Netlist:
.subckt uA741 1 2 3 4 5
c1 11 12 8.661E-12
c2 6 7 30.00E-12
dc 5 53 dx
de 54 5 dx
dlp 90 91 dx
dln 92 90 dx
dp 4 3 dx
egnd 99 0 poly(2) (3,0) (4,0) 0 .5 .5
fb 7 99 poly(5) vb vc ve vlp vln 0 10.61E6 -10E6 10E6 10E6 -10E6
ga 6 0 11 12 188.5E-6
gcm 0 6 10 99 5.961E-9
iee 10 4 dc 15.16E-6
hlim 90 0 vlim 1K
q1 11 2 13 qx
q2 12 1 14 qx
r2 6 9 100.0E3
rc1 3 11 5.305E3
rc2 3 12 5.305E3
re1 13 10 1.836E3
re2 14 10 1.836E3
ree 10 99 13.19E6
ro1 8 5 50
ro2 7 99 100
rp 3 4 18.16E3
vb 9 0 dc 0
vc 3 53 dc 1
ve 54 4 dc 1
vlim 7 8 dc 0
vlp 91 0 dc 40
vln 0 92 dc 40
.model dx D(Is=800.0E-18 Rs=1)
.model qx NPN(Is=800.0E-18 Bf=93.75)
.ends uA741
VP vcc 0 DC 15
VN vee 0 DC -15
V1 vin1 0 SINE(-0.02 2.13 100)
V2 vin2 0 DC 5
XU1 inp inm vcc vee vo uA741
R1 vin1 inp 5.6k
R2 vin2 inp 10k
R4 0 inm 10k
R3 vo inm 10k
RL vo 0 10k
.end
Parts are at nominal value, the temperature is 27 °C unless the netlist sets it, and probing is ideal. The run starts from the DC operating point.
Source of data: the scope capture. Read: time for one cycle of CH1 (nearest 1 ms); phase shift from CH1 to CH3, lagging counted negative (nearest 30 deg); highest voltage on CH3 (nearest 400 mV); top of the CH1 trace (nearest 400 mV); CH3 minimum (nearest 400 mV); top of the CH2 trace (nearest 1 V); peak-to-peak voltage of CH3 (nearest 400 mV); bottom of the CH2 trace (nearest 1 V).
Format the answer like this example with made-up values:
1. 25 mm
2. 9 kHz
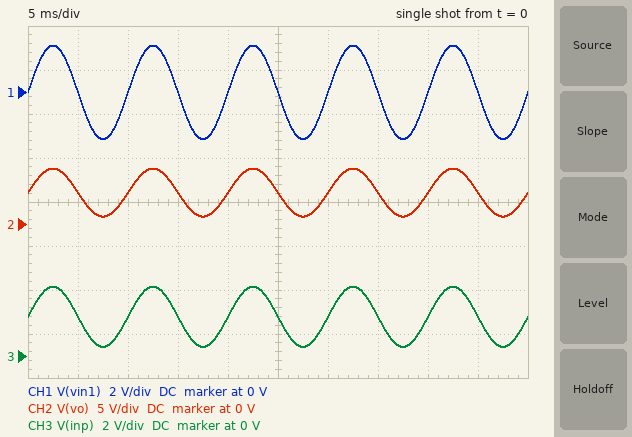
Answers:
1. 10 ms
2. 0 deg
3. 3.2 V
4. 2.0 V
5. 400 mV
6. 6 V
7. 2.8 V
8. 1 V
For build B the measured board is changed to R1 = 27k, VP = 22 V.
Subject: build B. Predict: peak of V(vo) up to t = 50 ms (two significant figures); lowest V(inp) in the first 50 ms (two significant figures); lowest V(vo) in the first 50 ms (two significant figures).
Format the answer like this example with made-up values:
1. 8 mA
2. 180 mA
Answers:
1. 8.4 V
2. 3.1 V
3. 6.1 V
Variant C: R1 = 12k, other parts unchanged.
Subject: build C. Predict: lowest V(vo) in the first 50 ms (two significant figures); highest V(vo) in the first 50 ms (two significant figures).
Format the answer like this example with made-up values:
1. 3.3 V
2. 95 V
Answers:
1. 3.5 V
2. 7.4 V
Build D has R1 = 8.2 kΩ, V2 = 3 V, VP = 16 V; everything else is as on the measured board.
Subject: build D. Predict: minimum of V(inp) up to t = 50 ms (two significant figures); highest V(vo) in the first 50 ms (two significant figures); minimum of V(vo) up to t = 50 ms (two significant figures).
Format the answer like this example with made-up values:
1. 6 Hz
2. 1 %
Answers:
1. 170 mV
2. 5.0 V
3. 340 mV
